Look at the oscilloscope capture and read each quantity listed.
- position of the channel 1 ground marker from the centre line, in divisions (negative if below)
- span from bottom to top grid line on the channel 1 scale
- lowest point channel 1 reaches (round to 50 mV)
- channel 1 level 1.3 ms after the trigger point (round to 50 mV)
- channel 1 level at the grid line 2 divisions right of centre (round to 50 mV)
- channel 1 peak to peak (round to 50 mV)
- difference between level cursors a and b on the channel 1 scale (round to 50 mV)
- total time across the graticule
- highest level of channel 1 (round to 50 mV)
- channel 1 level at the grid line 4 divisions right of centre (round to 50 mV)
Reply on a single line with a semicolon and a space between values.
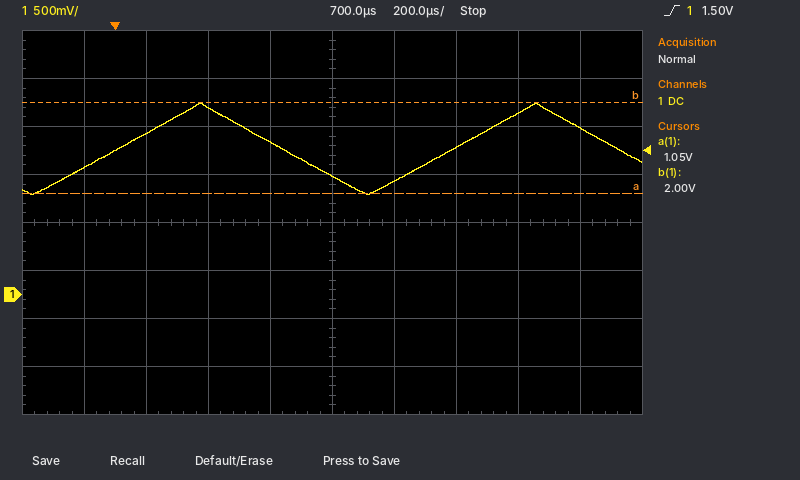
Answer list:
-1.5 div; 4 V; 1.05 V; 1.90 V; 1.55 V; 950 mV; 950 mV; 2 ms; 2.00 V; 1.75 V
